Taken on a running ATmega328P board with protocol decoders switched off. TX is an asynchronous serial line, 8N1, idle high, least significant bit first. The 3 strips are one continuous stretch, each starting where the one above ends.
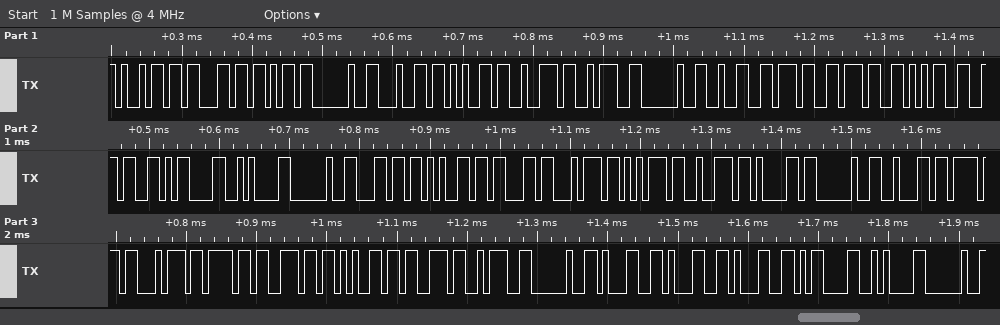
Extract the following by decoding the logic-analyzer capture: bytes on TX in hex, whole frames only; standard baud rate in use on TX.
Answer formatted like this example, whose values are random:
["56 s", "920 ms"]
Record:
["69 63 6B 20 64 65 72 3A 20 32 37 37 35 36 0D 0A 20 6C 65 63 74 75 72 61 20 62 6F 74 6F 6E 65 73 3A 20 31 31 31 0D 0A 20", "115200 baud"]
